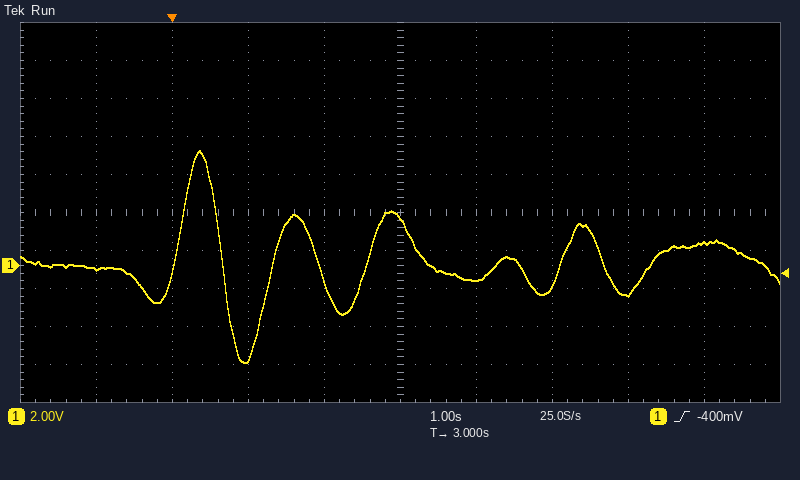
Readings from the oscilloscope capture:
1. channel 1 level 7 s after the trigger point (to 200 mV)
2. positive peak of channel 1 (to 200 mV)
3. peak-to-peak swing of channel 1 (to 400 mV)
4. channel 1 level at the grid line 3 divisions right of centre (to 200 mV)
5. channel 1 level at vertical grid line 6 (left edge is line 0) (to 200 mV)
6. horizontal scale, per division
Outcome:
1.2 V
6.0 V
11.2 V
-1.4 V
-800 mV
1 s
